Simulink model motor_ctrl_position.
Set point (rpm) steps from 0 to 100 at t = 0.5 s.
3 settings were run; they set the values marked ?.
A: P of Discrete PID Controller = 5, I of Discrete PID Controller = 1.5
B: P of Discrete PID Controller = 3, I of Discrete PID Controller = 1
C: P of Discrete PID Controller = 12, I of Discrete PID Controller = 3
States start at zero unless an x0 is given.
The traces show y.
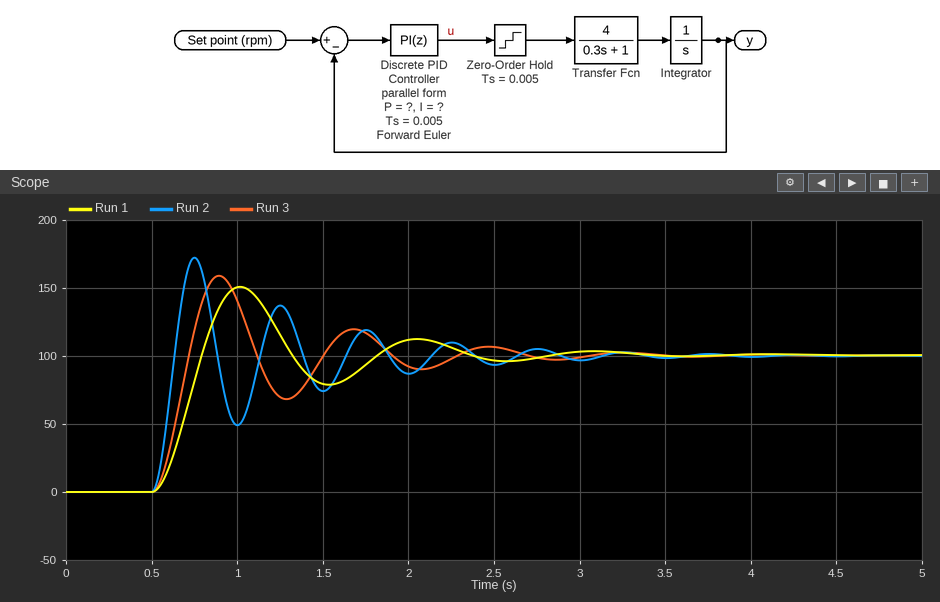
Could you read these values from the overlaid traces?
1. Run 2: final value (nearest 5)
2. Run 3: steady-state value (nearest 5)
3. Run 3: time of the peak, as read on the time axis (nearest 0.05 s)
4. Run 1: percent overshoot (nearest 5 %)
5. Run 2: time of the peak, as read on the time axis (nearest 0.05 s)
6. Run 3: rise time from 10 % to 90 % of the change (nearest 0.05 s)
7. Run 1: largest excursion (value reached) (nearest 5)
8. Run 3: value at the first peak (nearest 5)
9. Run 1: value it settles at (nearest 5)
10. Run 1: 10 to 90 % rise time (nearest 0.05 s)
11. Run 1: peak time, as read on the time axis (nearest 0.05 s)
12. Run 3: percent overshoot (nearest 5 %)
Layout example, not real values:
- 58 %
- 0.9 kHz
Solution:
- 100
- 100
- 0.90 s
- 50 %
- 0.75 s
- 0.15 s
- 150
- 160
- 100
- 0.20 s
- 1.00 s
- 60 %
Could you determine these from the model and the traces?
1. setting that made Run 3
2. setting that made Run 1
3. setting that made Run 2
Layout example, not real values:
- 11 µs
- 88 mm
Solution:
- A
- B
- C
